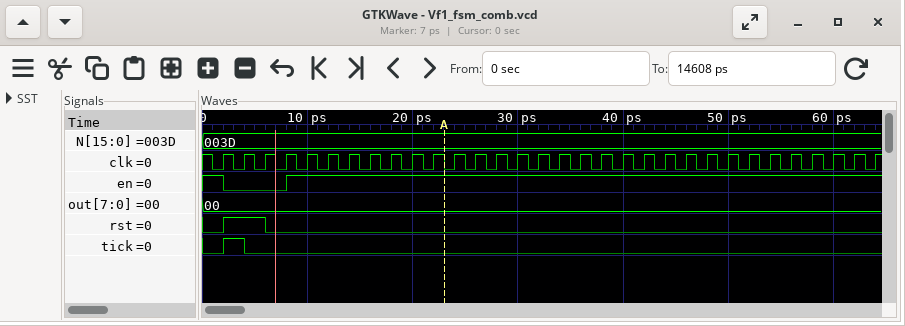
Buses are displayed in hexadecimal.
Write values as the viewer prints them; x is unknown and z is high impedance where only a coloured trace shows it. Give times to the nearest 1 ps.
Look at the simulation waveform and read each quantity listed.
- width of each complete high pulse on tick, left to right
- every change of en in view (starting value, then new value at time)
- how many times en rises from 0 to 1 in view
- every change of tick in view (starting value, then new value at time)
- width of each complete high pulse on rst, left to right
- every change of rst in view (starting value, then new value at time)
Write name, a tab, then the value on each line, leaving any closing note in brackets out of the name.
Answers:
width of each complete high pulse on tick, left to right	2 ps
every change of en in view	1, 0 at 2 ps, 1 at 8 ps
how many times en rises from 0 to 1 in view	1
every change of tick in view	0, 1 at 2 ps, 0 at 4 ps
width of each complete high pulse on rst, left to right	4 ps
every change of rst in view	0, 1 at 2 ps, 0 at 6 ps
